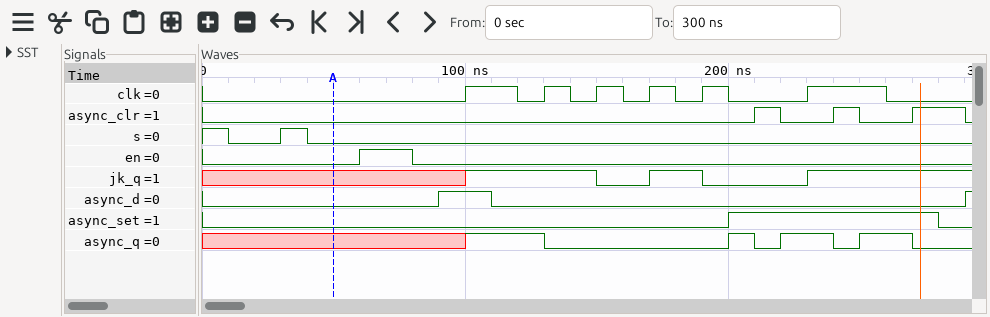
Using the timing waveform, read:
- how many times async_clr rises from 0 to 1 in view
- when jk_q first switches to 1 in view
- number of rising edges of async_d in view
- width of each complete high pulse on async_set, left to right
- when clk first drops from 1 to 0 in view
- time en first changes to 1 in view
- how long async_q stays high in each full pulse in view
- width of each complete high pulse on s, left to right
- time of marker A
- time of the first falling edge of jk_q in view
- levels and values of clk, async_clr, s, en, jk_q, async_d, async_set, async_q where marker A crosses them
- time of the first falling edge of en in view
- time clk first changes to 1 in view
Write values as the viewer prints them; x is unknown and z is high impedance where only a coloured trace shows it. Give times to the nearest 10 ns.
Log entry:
3
100 ns
2
80 ns
120 ns
60 ns
10 ns, 20 ns, 20 ns
10 ns
50 ns
150 ns
clk=0, async_clr=0, s=0, en=0, jk_q=x, async_d=0, async_set=0, async_q=x
80 ns
100 ns
